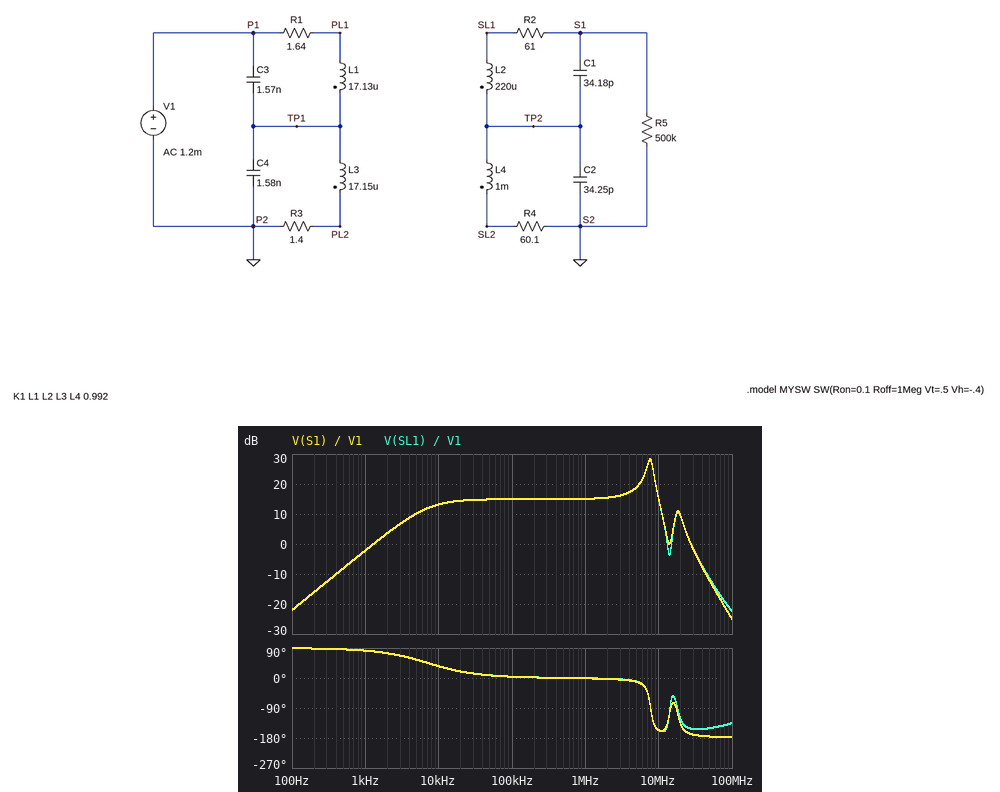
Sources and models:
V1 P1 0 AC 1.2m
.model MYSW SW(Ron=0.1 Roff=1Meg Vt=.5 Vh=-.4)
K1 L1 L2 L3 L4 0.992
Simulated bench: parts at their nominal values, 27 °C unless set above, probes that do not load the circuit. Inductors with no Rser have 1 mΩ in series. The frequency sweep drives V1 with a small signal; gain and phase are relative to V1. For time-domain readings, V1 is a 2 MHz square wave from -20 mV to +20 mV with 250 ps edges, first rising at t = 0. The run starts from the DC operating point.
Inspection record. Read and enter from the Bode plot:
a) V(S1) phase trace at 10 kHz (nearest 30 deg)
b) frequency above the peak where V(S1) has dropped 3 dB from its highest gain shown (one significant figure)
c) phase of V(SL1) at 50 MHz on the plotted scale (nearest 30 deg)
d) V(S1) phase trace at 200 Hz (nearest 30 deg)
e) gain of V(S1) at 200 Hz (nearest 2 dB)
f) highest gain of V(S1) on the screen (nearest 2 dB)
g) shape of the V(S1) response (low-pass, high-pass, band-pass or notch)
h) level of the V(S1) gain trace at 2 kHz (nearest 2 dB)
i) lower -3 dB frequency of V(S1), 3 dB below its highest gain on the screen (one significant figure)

30 deg
8 MHz
-150 deg
90 deg
-16 dB
28 dB
band-pass
4 dB
7 MHz
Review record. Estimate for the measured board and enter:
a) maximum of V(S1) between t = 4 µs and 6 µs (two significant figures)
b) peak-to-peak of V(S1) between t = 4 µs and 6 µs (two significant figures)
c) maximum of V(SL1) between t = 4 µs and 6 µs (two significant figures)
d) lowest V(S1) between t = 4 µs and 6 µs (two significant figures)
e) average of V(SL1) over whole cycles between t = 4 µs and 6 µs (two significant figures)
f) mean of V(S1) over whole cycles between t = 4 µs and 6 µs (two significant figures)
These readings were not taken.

310 mV
440 mV
310 mV
-130 mV
90 mV
90 mV
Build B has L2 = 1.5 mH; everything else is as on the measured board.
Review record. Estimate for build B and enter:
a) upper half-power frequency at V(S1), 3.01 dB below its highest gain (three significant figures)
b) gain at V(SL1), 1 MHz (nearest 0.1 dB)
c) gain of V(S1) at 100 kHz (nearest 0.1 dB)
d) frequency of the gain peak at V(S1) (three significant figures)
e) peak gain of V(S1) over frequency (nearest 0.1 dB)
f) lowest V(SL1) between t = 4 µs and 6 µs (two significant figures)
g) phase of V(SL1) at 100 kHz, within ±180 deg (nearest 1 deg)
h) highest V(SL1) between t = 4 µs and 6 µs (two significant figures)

6.51 MHz
18.8 dB
18.5 dB
5.90 MHz
31.4 dB
-400 mV
4 deg
670 mV
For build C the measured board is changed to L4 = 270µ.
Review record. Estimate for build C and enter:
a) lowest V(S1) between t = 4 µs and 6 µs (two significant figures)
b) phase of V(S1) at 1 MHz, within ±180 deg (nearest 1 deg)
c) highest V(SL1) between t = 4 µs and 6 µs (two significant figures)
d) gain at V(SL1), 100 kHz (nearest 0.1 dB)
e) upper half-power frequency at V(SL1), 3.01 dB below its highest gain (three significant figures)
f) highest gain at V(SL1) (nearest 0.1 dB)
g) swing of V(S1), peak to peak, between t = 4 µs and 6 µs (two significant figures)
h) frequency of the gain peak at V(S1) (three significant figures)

-120 mV
-1 deg
240 mV
11.5 dB
15.0 MHz
23.8 dB
370 mV
13.5 MHz
